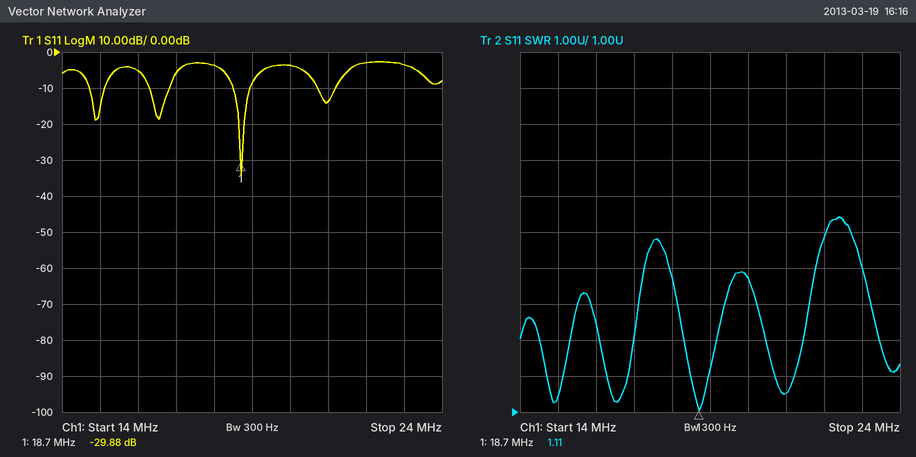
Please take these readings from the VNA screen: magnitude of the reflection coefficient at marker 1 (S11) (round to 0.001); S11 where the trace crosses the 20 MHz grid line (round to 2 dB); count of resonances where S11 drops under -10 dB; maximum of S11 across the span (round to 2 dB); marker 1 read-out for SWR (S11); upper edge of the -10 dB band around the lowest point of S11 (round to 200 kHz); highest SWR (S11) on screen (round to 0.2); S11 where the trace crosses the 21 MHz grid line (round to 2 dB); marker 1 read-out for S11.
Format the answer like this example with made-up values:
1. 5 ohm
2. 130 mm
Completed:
1. 0.032
2. -4 dB
3. 4
4. -2 dB
5. 1.11
6. 19.0 MHz
7. 6.4
8. -14 dB
9. -29.88 dB
